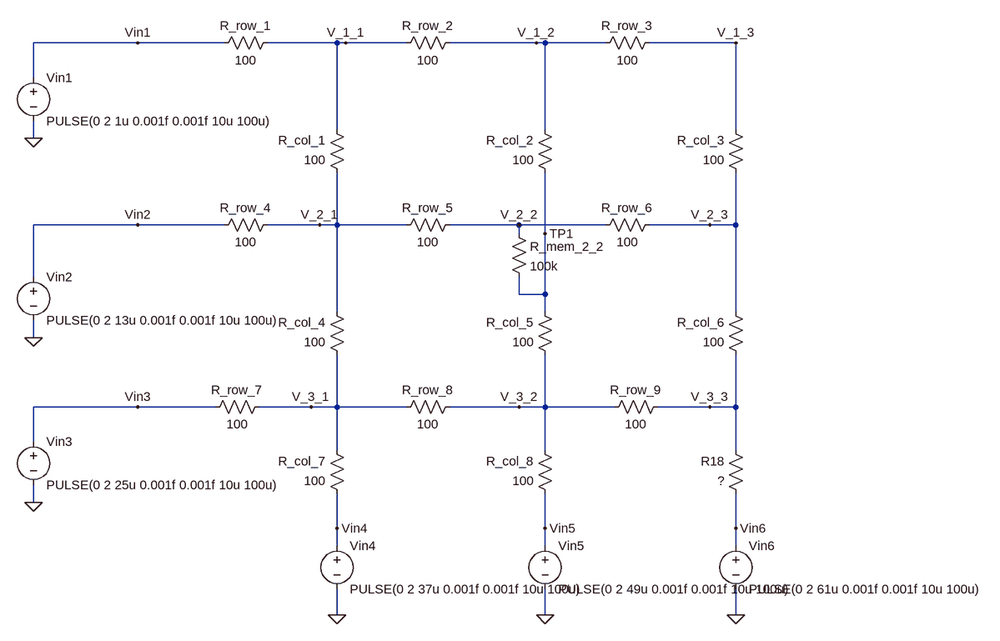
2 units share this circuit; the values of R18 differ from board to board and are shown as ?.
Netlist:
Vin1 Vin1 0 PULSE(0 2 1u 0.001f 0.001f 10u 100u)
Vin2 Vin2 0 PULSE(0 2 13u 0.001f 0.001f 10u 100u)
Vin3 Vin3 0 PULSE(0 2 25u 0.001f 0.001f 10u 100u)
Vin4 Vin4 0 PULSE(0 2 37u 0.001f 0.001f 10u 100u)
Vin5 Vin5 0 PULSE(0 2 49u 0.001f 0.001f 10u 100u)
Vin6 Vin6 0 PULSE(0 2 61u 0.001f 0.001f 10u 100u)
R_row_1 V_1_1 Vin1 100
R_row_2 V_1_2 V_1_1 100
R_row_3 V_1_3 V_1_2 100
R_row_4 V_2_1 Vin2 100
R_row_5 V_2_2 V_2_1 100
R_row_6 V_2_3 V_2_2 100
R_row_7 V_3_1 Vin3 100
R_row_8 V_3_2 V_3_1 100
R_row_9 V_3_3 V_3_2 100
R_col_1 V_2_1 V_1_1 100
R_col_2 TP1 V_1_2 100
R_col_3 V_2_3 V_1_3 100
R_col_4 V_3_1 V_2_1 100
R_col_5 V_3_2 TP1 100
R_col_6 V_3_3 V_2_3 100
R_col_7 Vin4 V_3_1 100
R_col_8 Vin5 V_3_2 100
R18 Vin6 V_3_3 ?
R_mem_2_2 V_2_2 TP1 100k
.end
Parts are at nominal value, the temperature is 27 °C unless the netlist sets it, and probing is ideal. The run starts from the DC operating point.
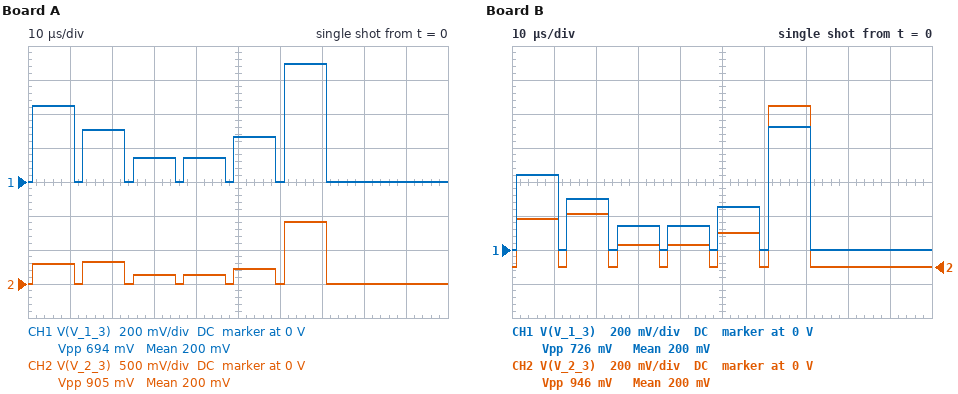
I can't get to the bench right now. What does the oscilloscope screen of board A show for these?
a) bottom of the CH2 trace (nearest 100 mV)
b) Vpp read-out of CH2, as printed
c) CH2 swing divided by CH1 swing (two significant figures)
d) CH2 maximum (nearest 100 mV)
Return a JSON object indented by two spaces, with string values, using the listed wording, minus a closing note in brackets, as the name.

{
  "bottom of the CH2 trace": "0 V",
  "Vpp read-out of CH2, as printed": "905 mV",
  "CH2 swing divided by CH1 swing": "1.3",
  "CH2 maximum": "900 mV"
}
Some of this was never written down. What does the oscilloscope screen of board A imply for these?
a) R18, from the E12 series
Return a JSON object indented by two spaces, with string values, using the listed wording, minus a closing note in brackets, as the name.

{
  "R18, from the E12 series": "39 Ω"
}
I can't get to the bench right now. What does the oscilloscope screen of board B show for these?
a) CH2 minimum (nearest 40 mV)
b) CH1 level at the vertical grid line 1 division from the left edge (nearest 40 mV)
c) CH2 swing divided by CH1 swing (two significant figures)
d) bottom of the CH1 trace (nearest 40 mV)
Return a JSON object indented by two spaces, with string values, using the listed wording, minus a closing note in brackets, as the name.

{
  "CH2 minimum": "0 V",
  "CH1 level at the vertical grid line 1 division from the left edge": "440 mV",
  "CH2 swing divided by CH1 swing": "1.3",
  "bottom of the CH1 trace": "0 V"
}
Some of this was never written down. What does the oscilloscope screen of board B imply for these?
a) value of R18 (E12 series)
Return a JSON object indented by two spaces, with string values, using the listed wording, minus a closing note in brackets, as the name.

{
  "value of R18": "33 Ω"
}
